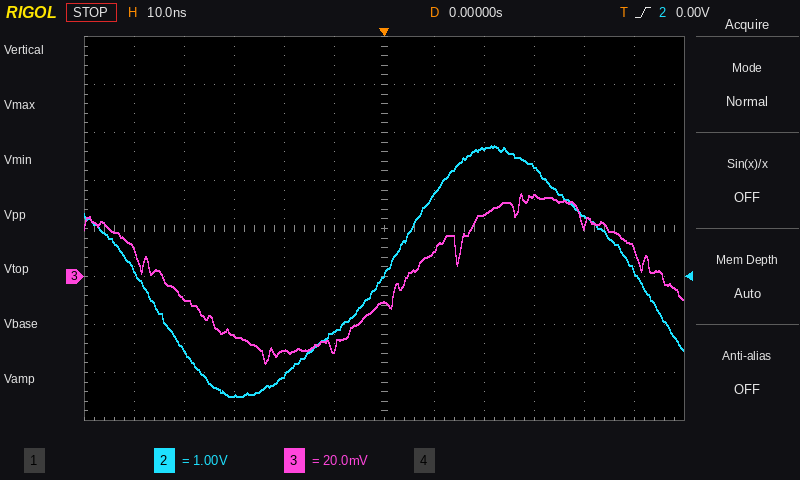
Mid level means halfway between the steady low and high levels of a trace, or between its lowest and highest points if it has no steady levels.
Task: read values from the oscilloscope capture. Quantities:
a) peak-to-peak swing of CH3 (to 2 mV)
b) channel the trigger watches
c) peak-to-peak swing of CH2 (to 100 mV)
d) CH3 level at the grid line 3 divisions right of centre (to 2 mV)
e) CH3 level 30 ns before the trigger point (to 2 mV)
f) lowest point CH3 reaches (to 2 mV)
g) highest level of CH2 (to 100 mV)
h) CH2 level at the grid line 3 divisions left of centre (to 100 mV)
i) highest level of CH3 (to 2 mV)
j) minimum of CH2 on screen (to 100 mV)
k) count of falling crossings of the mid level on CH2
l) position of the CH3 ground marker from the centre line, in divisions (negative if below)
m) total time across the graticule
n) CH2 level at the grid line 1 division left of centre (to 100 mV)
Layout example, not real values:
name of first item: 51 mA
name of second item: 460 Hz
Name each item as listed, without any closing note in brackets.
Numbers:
peak-to-peak swing of CH3: 70 mV
channel the trigger watches: CH2
peak-to-peak swing of CH2: 5.2 V
CH3 level at the grid line 3 divisions right of centre: 34 mV
CH3 level 30 ns before the trigger point: -24 mV
lowest point CH3 reaches: -36 mV
highest level of CH2: 2.7 V
CH2 level at the grid line 3 divisions left of centre: -2.5 V
highest level of CH3: 34 mV
minimum of CH2 on screen: -2.5 V
count of falling crossings of the mid level on CH2: 2
position of the CH3 ground marker from the centre line, in divisions: -1.0 div
total time across the graticule: 120 ns
CH2 level at the grid line 1 division left of centre: -1.1 V
